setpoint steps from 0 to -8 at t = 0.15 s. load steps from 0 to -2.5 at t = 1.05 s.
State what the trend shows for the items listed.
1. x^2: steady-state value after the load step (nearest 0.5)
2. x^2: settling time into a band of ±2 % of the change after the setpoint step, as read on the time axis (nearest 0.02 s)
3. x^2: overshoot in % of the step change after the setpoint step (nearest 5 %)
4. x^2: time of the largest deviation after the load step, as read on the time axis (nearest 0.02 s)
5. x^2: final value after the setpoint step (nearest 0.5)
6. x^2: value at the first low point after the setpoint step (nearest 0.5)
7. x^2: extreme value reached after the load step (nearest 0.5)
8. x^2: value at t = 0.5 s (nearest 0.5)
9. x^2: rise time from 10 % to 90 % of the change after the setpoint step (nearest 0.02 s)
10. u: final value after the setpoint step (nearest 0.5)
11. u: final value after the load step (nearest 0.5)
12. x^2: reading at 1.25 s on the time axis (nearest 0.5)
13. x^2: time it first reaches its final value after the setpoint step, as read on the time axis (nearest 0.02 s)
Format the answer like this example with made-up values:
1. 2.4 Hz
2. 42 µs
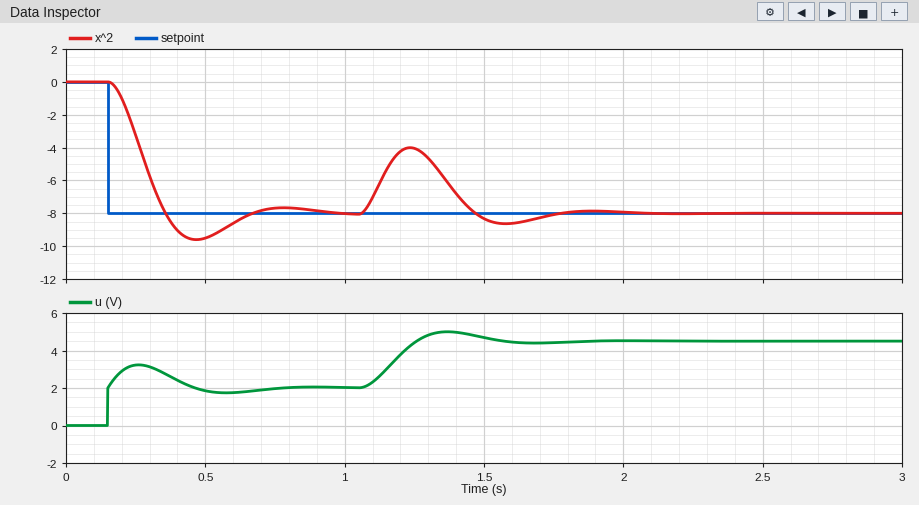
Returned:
1. -8.0
2. 0.90 s
3. 20 %
4. 1.24 s
5. -8.0
6. -9.5
7. -4.0
8. -9.5
9. 0.14 s
10. 2.0
11. 4.5
12. -4.0
13. 0.36 s
